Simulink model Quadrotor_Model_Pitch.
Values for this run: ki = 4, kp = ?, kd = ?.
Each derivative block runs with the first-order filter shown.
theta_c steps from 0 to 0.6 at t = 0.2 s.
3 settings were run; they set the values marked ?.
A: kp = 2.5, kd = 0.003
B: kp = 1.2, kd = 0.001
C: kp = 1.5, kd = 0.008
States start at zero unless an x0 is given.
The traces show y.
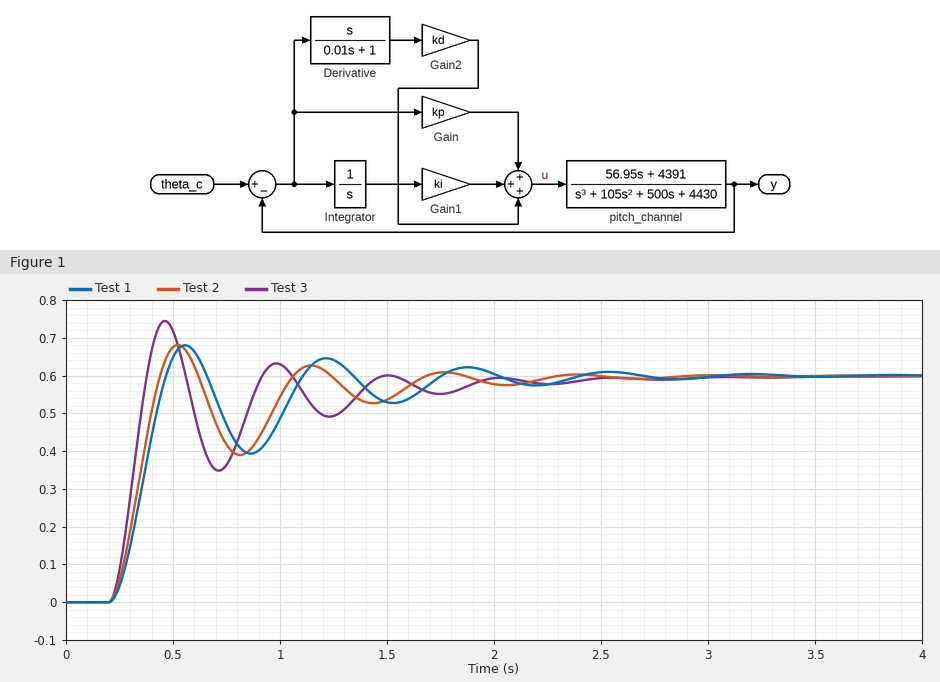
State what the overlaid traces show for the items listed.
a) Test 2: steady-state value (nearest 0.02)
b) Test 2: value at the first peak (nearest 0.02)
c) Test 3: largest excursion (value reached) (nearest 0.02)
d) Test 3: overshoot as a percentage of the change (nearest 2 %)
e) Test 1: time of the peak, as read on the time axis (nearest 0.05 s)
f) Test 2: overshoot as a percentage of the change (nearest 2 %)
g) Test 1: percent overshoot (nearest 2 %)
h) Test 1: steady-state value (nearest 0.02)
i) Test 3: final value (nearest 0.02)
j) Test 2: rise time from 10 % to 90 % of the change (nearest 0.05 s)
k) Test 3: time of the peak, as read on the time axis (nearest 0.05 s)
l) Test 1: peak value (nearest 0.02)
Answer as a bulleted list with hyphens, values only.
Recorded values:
- 0.60
- 0.68
- 0.74
- 24 %
- 0.55 s
- 14 %
- 14 %
- 0.60
- 0.60
- 0.15 s
- 0.45 s
- 0.68
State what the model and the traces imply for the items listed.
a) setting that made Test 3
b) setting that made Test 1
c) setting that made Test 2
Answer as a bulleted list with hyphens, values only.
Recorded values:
- A
- B
- C
